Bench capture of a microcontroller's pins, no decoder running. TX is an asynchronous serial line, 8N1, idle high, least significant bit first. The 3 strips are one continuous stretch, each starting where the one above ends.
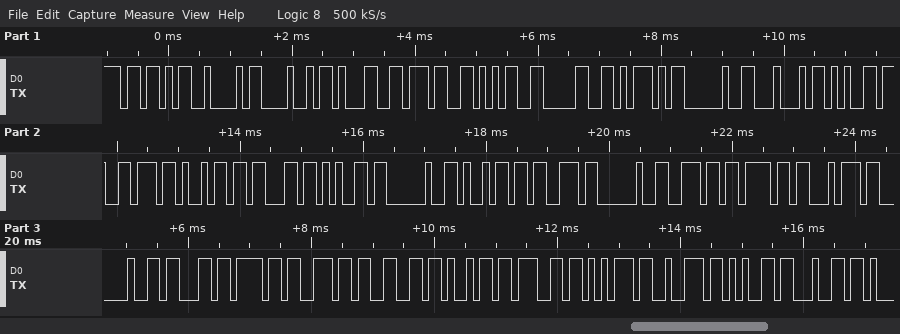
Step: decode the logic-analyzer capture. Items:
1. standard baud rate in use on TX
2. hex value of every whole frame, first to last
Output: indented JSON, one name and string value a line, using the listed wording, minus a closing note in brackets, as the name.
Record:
{
  "standard baud rate in use on TX": "9600 baud",
  "hex value of every whole frame, first to last": "5B 42 48 31 37 35 30 5D 20 44 65 76 69 63 65 20 69 73 20 6E 6F 74 20 63 6F 6E 66 69 67 75 72 65 64"
}
